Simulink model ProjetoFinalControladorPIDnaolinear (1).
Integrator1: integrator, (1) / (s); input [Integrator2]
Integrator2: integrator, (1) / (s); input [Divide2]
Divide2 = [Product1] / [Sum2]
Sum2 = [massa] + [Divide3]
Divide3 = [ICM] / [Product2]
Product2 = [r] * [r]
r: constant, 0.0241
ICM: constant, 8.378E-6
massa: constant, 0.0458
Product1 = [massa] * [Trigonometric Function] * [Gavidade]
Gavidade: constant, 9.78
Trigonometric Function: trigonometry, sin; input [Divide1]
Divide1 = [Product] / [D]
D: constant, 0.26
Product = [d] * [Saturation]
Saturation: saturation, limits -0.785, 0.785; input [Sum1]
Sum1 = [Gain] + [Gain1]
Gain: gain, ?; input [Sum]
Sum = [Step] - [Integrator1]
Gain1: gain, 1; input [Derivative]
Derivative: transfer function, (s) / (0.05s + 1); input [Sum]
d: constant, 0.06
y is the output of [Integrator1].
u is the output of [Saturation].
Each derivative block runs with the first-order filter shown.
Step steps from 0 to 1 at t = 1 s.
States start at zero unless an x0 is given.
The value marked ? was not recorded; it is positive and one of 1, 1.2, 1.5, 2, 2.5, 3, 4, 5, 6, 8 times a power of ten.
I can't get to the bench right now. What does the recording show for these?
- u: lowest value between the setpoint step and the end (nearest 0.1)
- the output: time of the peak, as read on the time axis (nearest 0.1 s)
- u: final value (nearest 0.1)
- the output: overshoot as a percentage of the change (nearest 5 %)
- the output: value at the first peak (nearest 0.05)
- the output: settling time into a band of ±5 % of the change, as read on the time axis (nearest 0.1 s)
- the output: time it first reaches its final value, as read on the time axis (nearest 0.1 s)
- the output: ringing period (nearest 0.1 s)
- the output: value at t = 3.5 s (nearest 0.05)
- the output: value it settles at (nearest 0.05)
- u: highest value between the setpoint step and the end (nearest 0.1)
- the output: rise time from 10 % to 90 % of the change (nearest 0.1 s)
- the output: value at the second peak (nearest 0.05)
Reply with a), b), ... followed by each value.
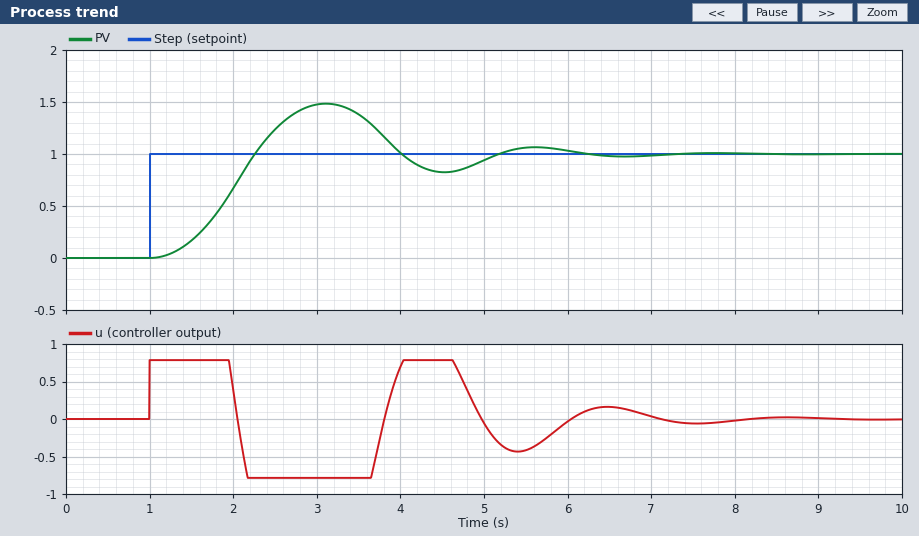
a) -0.8
b) 3.1 s
c) 0.0
d) 50 %
e) 1.50
f) 5.9 s
g) 2.3 s
h) 2.5 s
i) 1.40
j) 1.00
k) 0.8
l) 0.8 s
m) 1.05
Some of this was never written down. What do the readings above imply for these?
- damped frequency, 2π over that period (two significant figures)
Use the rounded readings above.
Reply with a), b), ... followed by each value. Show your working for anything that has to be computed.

a) 2π / 2.5 = 2.5 rad/s
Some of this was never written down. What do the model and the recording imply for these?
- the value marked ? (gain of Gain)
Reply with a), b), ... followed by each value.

a) 5
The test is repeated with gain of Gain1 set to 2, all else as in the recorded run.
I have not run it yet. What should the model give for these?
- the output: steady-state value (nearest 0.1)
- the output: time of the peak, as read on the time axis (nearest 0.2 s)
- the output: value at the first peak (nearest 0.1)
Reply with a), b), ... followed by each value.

a) 1.0
b) 2.8 s
c) 1.1
